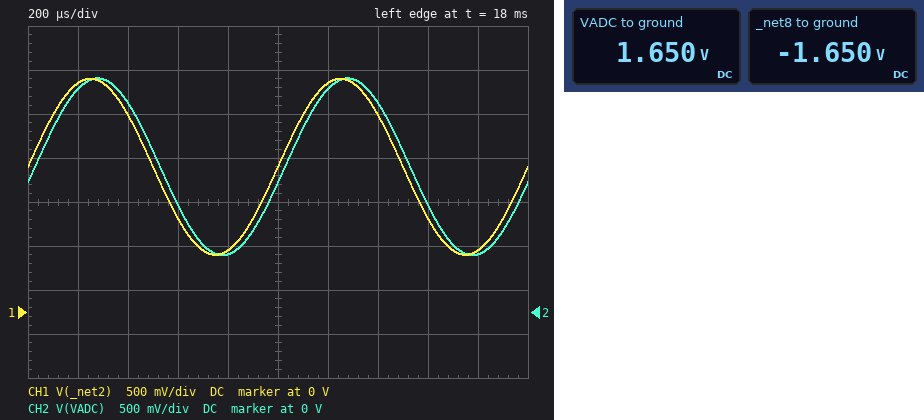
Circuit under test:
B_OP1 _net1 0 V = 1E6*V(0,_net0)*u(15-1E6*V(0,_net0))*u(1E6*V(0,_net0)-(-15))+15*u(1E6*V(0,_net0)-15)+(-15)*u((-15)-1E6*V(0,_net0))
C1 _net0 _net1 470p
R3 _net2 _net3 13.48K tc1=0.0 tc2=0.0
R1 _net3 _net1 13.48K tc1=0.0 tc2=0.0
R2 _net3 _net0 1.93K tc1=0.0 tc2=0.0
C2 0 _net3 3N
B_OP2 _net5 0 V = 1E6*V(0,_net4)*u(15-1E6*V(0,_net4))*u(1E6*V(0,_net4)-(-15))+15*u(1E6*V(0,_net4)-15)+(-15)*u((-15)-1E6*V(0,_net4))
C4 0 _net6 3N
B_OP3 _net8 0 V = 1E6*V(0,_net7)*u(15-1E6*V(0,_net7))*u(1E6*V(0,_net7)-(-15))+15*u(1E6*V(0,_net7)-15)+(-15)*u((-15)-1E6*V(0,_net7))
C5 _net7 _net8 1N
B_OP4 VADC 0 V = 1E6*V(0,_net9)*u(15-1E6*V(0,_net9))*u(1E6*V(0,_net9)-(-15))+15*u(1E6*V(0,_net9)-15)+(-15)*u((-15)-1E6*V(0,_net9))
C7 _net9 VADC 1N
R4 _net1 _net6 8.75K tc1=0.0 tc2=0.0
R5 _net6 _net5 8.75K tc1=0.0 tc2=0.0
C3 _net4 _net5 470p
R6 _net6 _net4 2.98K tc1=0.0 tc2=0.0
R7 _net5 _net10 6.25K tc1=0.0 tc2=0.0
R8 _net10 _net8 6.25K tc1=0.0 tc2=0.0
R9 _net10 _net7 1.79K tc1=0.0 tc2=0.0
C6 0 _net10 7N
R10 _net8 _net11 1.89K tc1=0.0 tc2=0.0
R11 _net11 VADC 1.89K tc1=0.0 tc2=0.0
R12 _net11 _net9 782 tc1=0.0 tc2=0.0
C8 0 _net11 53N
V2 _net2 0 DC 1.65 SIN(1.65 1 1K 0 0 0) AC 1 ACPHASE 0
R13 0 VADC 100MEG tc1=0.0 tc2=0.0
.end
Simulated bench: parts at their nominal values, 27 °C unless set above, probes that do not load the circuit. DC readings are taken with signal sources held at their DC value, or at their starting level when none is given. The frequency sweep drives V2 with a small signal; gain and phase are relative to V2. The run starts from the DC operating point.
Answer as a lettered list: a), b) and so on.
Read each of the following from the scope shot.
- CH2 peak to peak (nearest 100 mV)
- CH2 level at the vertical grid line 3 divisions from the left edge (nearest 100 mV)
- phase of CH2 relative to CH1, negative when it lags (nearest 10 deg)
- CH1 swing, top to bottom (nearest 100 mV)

a) 2.0 V
b) 1.2 V
c) -10 deg
d) 2.0 V
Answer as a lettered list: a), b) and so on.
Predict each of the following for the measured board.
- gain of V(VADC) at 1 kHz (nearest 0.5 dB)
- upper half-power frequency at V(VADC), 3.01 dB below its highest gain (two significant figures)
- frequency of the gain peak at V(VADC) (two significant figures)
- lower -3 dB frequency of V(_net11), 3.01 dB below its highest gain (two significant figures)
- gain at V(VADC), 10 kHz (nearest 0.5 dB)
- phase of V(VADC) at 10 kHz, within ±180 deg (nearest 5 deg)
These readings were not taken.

a) 0 dB
b) 19 kHz
c) 16 kHz
d) 14 kHz
e) 4.0 dB
f) -115 deg
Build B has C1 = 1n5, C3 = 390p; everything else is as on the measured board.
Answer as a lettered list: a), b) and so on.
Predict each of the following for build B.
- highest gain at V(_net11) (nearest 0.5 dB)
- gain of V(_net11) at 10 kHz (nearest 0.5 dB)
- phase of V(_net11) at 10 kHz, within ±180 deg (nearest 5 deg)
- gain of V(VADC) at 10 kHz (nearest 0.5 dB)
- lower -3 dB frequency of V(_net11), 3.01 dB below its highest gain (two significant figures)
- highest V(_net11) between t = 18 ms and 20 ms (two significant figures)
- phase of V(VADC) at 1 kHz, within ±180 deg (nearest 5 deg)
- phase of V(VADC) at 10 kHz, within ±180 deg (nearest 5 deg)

a) -21.5 dB
b) -27.0 dB
c) 115 deg
d) -1.0 dB
e) 12 kHz
f) 4.9 mV
g) -15 deg
h) -155 deg
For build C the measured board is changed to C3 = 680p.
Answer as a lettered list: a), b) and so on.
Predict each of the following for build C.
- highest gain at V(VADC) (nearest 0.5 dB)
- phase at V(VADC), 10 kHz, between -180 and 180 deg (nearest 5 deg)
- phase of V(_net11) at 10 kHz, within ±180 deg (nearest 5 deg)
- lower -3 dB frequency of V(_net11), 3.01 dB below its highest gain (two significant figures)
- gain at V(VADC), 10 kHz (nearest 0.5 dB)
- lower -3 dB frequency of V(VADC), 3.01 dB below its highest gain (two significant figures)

a) 6.5 dB
b) -130 deg
c) 140 deg
d) 13 kHz
e) 3.5 dB
f) 10 kHz
